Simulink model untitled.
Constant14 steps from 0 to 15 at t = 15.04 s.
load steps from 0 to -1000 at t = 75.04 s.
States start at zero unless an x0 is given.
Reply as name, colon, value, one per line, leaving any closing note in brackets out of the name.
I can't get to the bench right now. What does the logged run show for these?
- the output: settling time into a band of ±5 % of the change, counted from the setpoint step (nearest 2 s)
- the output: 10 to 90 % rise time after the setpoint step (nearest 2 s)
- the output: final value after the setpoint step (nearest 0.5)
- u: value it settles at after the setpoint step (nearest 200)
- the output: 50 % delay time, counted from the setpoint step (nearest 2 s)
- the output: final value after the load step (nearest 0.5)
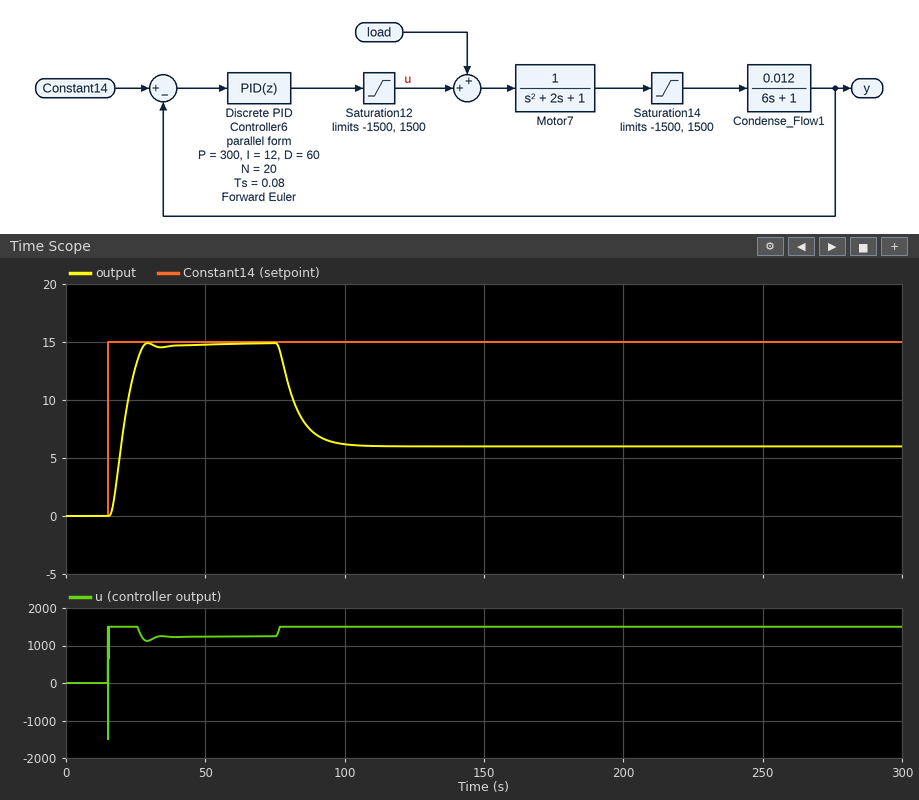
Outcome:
the output: settling time into a band of ±5 % of the change, counted from the setpoint step: 12 s
the output: 10 to 90 % rise time after the setpoint step: 8 s
the output: final value after the setpoint step: 15.0
u: value it settles at after the setpoint step: 1200
the output: 50 % delay time, counted from the setpoint step: 6 s
the output: final value after the load step: 6.0
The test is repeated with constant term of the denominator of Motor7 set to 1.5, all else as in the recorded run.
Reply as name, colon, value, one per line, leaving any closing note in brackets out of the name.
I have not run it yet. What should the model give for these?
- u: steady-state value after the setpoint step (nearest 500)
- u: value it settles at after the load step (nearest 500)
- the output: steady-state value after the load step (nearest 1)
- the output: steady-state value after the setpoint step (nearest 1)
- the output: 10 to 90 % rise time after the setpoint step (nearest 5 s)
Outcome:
u: steady-state value after the setpoint step: 1500
u: value it settles at after the load step: 1500
the output: steady-state value after the load step: 4
the output: steady-state value after the setpoint step: 12
the output: 10 to 90 % rise time after the setpoint step: 15 s
